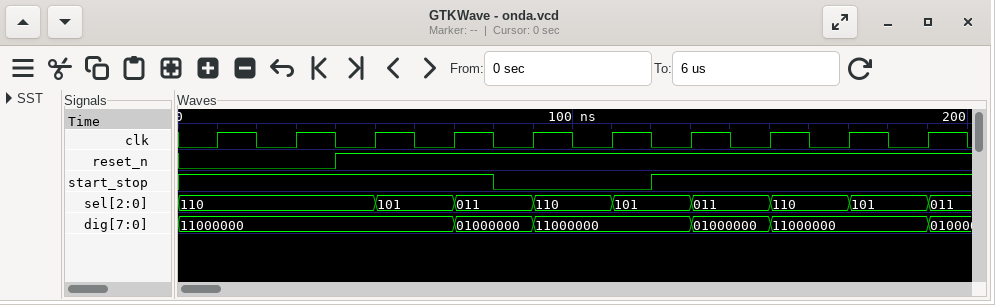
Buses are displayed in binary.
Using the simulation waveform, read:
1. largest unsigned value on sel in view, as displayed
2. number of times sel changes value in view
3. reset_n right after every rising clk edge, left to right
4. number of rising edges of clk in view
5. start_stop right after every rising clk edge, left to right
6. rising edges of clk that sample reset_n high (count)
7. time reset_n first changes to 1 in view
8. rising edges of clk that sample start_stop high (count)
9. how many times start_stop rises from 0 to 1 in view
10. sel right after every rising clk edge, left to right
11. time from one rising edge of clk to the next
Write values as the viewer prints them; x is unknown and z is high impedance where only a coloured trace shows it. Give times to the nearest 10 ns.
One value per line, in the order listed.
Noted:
110
8
0 0 1 1 1 1 1 1 1 1
10
1 1 1 1 0 0 1 1 1 1
8
40 ns
8
1
110, 110, 101, 011, 110, 101, 011, 110, 101, 011
20 ns
